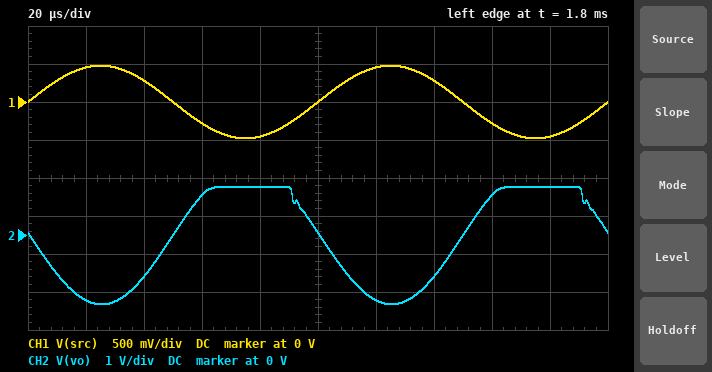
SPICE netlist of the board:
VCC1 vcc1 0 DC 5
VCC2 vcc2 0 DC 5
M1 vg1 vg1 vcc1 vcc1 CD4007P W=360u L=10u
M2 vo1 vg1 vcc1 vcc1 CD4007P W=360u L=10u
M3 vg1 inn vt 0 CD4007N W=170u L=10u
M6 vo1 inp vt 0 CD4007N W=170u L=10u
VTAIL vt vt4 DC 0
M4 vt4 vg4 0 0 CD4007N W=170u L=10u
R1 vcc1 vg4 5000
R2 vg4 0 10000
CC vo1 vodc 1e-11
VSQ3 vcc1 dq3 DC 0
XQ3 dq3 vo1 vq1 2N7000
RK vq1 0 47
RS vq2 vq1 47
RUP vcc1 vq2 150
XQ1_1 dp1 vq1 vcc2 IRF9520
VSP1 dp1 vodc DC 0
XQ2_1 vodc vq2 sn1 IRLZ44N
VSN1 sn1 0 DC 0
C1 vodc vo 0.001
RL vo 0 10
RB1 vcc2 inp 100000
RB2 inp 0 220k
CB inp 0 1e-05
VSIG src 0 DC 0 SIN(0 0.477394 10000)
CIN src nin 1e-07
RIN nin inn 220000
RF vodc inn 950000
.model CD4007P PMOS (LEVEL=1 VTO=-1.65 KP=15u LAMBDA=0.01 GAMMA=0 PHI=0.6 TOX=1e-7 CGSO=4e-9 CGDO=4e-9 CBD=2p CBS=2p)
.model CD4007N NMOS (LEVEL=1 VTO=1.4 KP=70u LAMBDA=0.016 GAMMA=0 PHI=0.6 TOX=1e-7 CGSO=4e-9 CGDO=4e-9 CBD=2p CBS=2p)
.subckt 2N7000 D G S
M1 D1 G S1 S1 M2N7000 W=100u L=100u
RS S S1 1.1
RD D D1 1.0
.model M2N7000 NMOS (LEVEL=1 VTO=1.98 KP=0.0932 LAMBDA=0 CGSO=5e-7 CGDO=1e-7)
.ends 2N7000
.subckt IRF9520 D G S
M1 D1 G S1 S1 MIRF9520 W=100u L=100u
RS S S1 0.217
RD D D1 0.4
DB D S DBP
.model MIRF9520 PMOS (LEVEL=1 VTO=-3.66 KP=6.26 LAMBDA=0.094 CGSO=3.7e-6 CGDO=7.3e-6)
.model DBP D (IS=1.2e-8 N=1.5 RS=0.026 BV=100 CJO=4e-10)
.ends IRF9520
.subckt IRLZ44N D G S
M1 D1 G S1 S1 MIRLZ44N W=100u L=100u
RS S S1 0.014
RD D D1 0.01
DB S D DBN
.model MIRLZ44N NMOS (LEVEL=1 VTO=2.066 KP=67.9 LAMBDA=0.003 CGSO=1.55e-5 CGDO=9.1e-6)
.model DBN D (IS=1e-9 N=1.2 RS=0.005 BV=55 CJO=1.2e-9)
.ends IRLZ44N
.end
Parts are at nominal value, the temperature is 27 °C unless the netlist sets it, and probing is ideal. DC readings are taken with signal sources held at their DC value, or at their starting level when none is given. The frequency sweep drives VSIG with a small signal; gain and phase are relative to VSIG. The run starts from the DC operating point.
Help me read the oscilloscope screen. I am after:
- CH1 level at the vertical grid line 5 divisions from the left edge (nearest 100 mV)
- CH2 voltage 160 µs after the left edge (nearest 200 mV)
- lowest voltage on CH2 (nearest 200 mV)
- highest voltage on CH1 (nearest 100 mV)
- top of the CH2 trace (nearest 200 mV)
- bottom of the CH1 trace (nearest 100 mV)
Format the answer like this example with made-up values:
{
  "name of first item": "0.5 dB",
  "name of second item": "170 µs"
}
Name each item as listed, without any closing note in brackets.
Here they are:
{
  "CH1 level at the vertical grid line 5 divisions from the left edge": "0 V",
  "CH2 voltage 160 µs after the left edge": "1.0 V",
  "lowest voltage on CH2": "-1.8 V",
  "highest voltage on CH1": "500 mV",
  "top of the CH2 trace": "1.2 V",
  "bottom of the CH1 trace": "-500 mV"
}
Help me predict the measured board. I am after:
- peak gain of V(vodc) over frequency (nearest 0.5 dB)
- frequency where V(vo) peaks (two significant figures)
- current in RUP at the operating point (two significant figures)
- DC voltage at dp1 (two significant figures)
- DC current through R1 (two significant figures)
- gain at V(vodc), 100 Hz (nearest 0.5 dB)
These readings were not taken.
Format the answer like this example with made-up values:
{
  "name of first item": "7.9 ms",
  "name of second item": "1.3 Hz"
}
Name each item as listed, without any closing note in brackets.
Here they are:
{
  "peak gain of V(vodc) over frequency": "17.5 dB",
  "frequency where V(vo) peaks": "390 kHz",
  "current in RUP at the operating point": "19 mA",
  "DC voltage at dp1": "3.6 V",
  "DC current through R1": "330 µA",
  "gain at V(vodc), 100 Hz": "11.5 dB"
}
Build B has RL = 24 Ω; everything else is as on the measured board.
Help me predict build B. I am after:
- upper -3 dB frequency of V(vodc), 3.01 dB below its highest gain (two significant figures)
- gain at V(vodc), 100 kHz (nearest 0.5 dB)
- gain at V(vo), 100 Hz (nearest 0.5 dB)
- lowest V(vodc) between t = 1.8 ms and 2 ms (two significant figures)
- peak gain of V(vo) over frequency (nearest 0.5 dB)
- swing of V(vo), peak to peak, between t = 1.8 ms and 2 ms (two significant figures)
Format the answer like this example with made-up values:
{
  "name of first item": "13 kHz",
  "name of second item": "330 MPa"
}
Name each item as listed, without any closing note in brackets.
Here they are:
{
  "upper -3 dB frequency of V(vodc), 3.01 dB below its highest gain": "470 kHz",
  "gain at V(vodc), 100 kHz": "12.5 dB",
  "gain at V(vo), 100 Hz": "12.0 dB",
  "lowest V(vodc) between t = 1.8 ms and 2 ms": "1.7 V",
  "peak gain of V(vo) over frequency": "19.5 dB",
  "swing of V(vo), peak to peak, between t = 1.8 ms and 2 ms": "3.3 V"
}
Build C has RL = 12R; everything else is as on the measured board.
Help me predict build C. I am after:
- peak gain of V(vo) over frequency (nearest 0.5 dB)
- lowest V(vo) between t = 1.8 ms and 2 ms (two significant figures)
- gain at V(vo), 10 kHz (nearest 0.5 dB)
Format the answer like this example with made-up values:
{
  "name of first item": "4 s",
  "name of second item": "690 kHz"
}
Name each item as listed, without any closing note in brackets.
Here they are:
{
  "peak gain of V(vo) over frequency": "18.0 dB",
  "lowest V(vo) between t = 1.8 ms and 2 ms": "-1.9 V",
  "gain at V(vo), 10 kHz": "12.0 dB"
}
